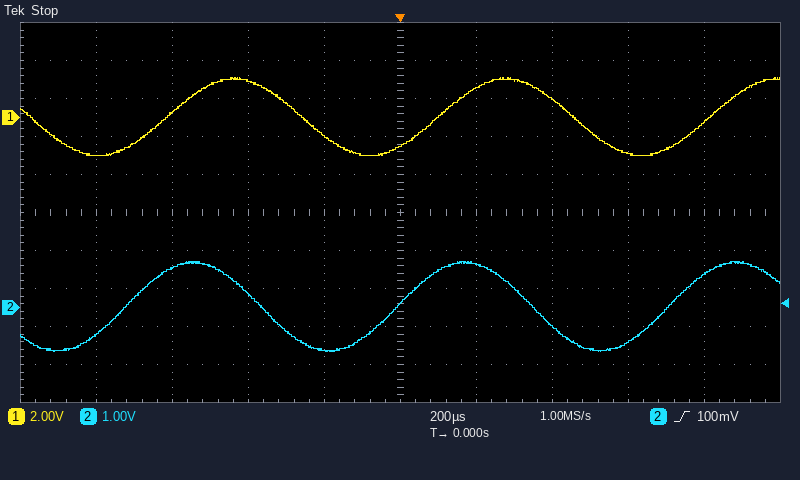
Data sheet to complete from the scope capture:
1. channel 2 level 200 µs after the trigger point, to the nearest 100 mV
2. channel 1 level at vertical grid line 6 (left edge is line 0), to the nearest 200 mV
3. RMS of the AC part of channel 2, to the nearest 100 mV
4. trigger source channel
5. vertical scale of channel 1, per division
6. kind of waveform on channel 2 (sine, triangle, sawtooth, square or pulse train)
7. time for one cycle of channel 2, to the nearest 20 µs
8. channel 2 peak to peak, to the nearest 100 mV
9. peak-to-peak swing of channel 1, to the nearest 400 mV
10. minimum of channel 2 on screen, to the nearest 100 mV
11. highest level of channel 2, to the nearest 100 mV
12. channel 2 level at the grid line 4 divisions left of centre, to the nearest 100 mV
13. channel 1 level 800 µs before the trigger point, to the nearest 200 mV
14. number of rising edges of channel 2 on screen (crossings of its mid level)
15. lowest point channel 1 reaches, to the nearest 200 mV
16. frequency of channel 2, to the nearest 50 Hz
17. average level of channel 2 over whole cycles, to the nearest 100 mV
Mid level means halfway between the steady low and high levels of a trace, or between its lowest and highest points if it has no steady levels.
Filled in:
1.1 V
1.6 V
800 mV
channel 2
2 V
sine
720 µs
2.4 V
4.0 V
-1.2 V
1.2 V
-700 mV
-2.0 V
3
-2.0 V
1.40 kHz
0.0 V
